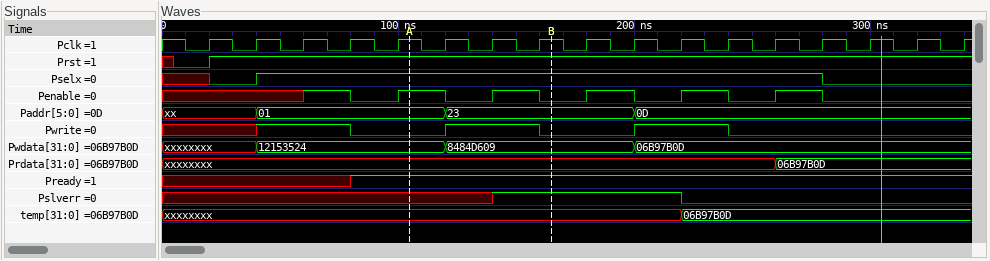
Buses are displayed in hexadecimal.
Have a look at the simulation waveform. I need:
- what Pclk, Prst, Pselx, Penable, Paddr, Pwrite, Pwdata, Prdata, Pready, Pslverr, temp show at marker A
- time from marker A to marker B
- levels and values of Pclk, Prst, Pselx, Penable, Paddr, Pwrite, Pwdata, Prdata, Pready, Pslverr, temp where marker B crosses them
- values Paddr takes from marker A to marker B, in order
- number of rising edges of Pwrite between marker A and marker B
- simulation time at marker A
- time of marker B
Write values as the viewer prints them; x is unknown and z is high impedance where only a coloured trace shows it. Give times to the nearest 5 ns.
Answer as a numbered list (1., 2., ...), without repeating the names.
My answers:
1. Pclk=1, Prst=1, Pselx=1, Penable=1, Paddr=01, Pwrite=0, Pwdata=12153524, Prdata=xxxxxxxx, Pready=1, Pslverr=x, temp=xxxxxxxx
2. 60 ns
3. Pclk=1, Prst=1, Pselx=1, Penable=0, Paddr=23, Pwrite=0, Pwdata=8484D609, Prdata=xxxxxxxx, Pready=1, Pslverr=1, temp=xxxxxxxx
4. 01, 23
5. 1
6. 105 ns
7. 165 ns
